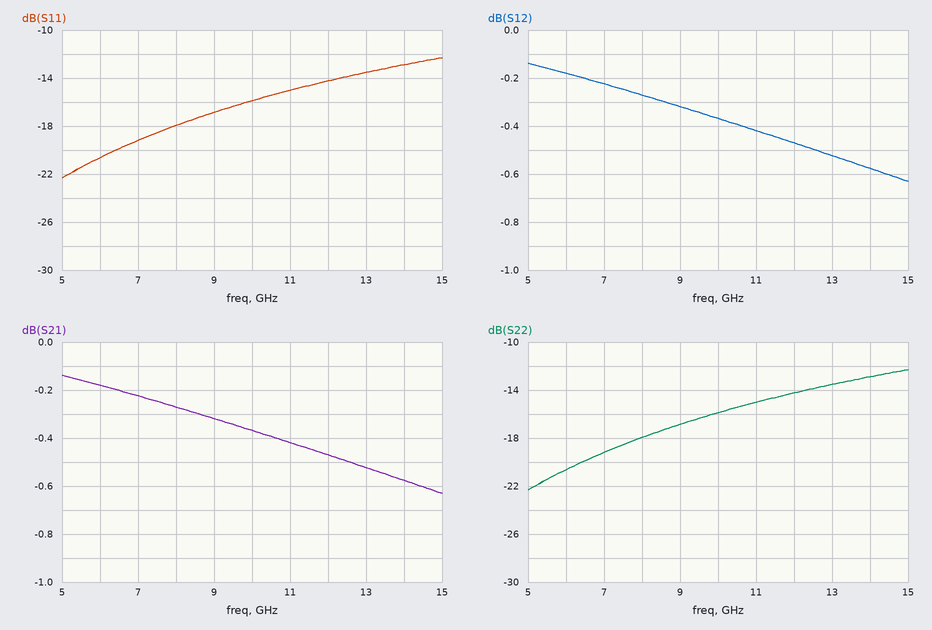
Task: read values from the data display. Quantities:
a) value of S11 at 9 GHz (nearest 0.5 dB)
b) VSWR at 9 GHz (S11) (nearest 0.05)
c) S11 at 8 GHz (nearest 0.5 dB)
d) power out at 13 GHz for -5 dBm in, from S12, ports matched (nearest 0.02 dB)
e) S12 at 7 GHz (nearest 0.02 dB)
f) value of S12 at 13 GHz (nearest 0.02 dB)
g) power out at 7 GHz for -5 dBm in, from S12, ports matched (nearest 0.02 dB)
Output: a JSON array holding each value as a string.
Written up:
["-17.0 dB", "1.35", "-18.0 dB", "-5.52 dBm", "-0.22 dB", "-0.52 dB", "-5.22 dBm"]
